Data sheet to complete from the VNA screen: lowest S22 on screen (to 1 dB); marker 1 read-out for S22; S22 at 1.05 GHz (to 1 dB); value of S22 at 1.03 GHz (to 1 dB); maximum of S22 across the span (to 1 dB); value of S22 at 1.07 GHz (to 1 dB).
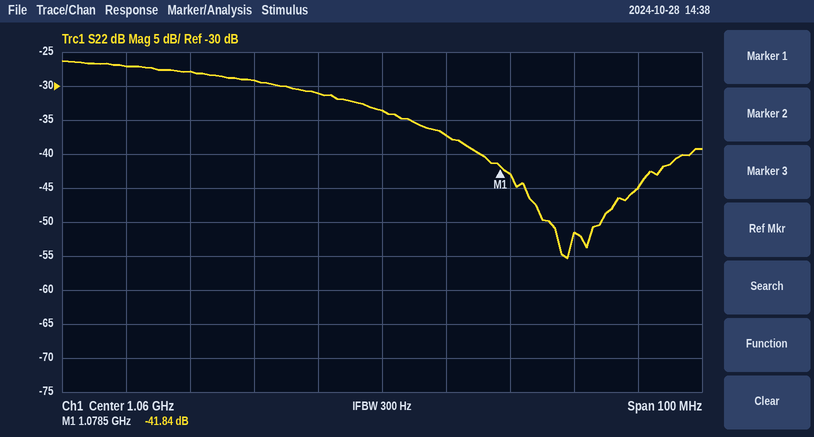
-55 dB
-41.84 dB
-31 dB
-28 dB
-26 dB
-37 dB
